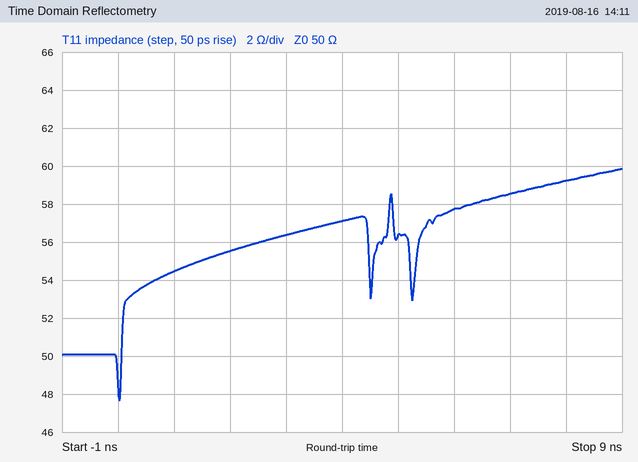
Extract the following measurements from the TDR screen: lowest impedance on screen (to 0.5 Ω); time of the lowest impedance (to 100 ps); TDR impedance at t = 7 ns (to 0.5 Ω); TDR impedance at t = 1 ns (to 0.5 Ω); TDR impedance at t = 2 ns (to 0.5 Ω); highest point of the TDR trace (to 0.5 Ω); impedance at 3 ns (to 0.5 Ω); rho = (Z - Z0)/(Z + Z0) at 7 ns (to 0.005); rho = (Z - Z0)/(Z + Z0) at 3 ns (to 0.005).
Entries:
47.5 Ω
0.0 ns
58.5 Ω
54.5 Ω
55.5 Ω
60.0 Ω
56.5 Ω
+0.080
+0.060
